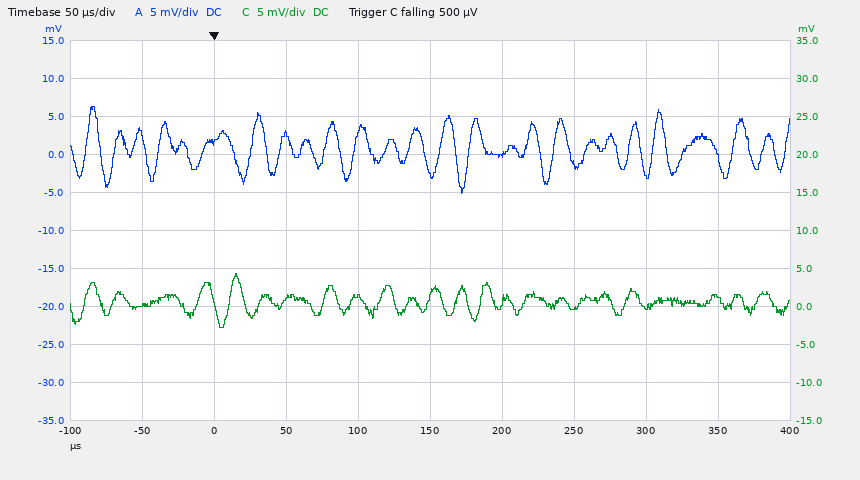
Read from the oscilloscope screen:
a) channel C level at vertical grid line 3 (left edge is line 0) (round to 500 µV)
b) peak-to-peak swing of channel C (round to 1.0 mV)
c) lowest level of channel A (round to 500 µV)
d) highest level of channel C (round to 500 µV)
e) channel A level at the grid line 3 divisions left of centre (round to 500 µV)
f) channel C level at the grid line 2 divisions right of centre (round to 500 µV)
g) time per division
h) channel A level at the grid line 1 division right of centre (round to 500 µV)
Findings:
1.0 mV
7.0 mV
-5.0 mV
4.5 mV
1.5 mV
0.0 mV
50 µs
0.0 mV
